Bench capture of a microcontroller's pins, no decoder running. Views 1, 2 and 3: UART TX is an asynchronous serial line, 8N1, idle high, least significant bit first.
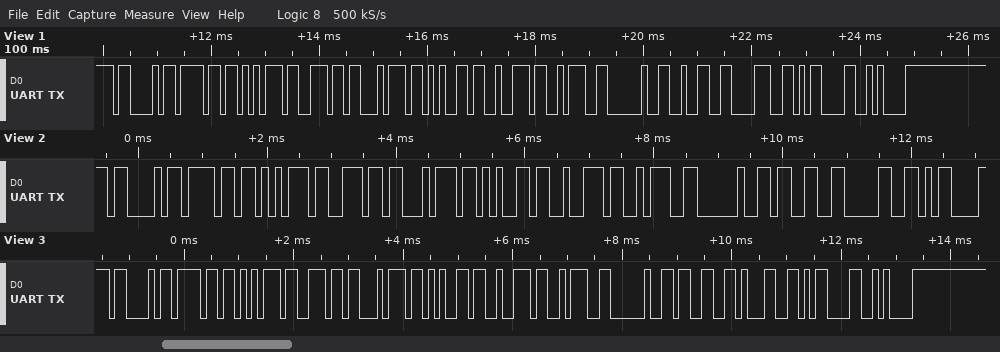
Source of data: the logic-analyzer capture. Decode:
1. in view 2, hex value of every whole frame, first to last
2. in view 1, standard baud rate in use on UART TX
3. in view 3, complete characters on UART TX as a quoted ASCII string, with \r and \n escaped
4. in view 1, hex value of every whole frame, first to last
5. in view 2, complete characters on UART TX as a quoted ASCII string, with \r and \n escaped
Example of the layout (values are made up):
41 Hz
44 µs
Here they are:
43 6F 75 6E 74 65 72 3A 20 33 30 0D
9600 baud
"Counter: 31\r\n"
43 6F 75 6E 74 65 72 3A 20 32 38 0D 0A
"Counter: 30\r"
